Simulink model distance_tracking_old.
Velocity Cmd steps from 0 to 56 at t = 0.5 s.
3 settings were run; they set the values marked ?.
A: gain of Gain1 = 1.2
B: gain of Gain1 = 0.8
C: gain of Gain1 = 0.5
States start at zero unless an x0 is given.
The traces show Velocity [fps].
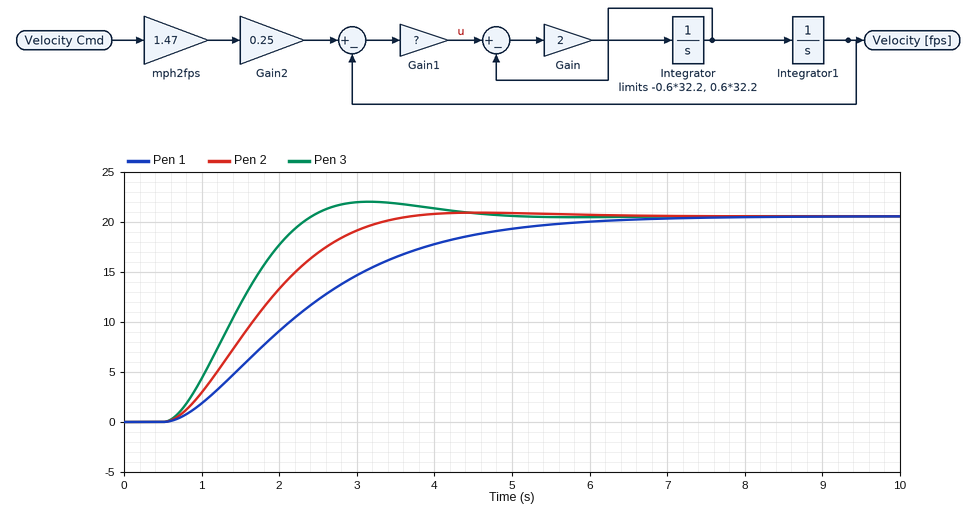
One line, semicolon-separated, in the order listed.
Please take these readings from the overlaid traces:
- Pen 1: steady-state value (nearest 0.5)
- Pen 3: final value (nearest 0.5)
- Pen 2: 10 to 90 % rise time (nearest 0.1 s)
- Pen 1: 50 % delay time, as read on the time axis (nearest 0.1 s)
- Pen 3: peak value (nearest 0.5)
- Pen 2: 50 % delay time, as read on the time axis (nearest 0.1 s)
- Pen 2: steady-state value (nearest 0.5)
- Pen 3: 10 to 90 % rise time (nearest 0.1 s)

20.5; 20.5; 1.9 s; 2.2 s; 22.0; 1.7 s; 20.5; 1.3 s
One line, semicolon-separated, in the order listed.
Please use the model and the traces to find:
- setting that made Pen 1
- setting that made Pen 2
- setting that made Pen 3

C; B; A
